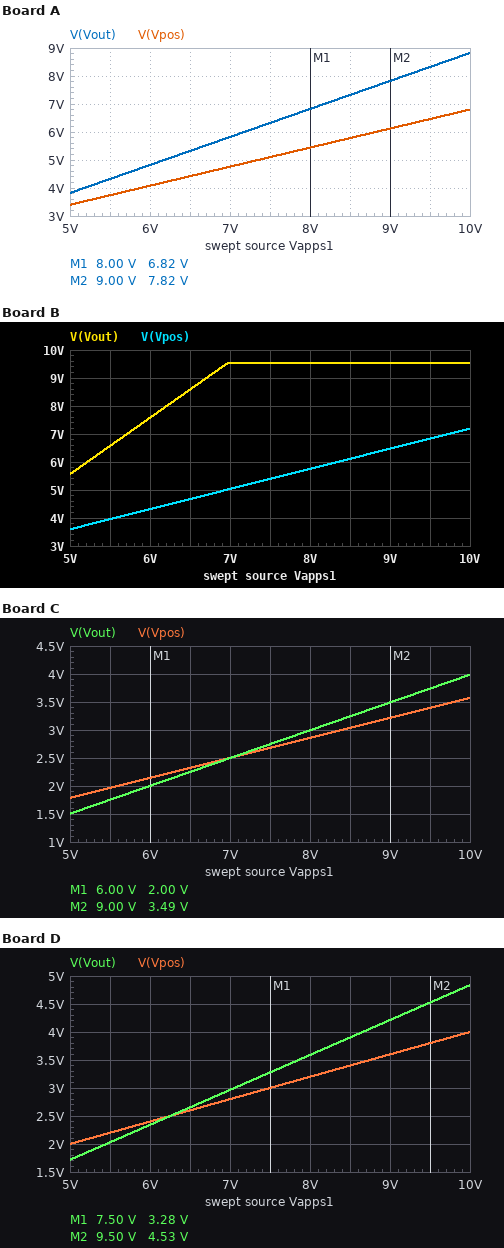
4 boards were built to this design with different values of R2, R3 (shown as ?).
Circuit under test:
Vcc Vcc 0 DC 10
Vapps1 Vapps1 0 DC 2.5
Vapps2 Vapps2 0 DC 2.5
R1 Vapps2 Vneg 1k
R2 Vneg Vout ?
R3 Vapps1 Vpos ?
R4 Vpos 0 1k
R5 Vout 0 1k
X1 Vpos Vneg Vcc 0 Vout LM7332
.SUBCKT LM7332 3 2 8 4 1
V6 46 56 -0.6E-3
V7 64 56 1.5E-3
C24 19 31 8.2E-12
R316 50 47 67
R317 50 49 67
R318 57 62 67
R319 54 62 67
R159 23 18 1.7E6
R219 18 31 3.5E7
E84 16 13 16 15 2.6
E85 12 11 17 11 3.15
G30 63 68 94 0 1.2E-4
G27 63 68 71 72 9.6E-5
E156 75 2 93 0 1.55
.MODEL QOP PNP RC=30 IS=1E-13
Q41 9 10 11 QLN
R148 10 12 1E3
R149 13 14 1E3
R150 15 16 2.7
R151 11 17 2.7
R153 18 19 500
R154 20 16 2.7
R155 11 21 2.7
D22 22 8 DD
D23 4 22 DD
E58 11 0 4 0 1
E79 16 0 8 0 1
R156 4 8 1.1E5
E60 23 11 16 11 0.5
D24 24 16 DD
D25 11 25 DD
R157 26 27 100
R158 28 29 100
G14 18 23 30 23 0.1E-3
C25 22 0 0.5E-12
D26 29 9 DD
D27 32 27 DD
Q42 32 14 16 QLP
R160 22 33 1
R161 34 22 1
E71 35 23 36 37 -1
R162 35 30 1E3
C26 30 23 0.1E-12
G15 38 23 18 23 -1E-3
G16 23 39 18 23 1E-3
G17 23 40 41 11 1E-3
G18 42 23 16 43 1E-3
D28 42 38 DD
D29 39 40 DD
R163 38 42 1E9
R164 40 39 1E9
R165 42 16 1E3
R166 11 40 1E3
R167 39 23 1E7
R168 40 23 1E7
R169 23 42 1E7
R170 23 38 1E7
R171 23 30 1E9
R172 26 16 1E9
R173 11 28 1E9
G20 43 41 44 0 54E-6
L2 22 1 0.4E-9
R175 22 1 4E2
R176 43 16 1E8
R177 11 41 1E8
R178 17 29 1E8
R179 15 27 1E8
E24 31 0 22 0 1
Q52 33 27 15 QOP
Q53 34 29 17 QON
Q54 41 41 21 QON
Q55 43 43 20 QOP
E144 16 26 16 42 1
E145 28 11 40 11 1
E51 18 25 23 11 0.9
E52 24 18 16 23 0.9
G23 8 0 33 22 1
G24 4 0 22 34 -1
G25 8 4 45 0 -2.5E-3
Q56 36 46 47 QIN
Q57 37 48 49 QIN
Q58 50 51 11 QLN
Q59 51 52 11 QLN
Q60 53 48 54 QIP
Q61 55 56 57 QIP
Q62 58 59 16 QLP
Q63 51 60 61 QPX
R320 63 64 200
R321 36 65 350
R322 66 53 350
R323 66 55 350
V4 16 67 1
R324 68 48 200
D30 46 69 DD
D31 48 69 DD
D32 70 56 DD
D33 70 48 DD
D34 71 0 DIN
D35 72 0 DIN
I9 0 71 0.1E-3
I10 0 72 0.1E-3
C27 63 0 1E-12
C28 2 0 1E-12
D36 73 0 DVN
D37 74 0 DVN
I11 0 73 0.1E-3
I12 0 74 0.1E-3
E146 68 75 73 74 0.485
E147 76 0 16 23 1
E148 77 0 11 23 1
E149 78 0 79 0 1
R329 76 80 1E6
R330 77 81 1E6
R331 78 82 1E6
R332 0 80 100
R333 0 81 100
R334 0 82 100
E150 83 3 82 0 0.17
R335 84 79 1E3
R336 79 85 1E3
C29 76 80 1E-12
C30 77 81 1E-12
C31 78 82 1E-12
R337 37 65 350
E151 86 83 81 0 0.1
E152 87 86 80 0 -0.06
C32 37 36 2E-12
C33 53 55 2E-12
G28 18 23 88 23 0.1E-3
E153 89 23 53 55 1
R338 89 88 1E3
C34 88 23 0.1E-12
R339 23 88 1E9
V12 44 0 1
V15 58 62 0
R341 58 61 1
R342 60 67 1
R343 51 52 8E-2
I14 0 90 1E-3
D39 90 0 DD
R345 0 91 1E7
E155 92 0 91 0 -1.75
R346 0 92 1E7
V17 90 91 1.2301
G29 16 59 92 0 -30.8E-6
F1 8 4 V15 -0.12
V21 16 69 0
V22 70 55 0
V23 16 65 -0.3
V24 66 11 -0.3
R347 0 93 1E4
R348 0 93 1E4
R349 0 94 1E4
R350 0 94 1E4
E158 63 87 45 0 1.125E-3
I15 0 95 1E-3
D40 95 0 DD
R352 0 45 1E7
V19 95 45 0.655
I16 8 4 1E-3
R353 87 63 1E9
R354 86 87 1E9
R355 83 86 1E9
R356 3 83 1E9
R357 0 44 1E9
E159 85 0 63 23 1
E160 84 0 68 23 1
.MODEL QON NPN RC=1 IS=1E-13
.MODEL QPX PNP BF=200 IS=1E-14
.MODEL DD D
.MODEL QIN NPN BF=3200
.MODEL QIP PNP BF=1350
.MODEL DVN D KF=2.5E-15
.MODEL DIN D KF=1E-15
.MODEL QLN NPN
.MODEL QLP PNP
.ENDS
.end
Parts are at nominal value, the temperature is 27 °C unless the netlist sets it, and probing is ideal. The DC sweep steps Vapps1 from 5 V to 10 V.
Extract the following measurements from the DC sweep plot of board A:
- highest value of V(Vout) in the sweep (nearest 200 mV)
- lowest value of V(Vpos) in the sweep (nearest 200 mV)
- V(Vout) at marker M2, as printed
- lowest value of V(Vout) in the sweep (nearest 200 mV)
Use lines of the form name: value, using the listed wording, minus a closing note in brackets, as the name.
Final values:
highest value of V(Vout) in the sweep: 8.8 V
lowest value of V(Vpos) in the sweep: 3.4 V
V(Vout) at marker M2, as printed: 7.82 V
lowest value of V(Vout) in the sweep: 3.8 V
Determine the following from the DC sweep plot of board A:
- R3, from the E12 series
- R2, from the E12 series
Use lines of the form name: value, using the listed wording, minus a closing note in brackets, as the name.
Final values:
R3, from the E12 series: 470 Ω
R2, from the E12 series: 470 Ω
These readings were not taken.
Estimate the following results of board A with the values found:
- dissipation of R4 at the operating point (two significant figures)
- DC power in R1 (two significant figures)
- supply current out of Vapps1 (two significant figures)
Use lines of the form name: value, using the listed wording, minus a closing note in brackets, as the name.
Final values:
dissipation of R4 at the operating point: 2.9 mW
DC power in R1: 640 µW
supply current out of Vapps1: 1.7 mA
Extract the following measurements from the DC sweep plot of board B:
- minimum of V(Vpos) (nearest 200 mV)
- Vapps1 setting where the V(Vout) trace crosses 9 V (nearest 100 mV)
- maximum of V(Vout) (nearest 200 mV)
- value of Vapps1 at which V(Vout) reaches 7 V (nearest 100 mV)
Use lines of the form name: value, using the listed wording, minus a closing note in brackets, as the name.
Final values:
minimum of V(Vpos): 3.6 V
Vapps1 setting where the V(Vout) trace crosses 9 V: 6.7 V
maximum of V(Vout): 9.6 V
value of Vapps1 at which V(Vout) reaches 7 V: 5.7 V
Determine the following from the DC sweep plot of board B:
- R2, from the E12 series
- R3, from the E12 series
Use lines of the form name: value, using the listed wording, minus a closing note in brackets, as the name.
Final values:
R2, from the E12 series: 1.8 kΩ
R3, from the E12 series: 390 Ω
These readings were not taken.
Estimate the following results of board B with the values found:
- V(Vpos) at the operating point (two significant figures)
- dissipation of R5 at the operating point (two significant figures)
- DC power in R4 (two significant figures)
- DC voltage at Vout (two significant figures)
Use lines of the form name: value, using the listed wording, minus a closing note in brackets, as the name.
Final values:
V(Vpos) at the operating point: 1.8 V
dissipation of R5 at the operating point: 280 µW
DC power in R4: 3.2 mW
DC voltage at Vout: 530 mV
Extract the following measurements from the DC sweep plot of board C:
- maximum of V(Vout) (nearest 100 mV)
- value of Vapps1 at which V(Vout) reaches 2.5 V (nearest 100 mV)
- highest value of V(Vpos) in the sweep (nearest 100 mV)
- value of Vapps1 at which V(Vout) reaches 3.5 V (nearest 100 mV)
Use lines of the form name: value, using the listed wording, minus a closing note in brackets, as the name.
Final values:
maximum of V(Vout): 4.0 V
value of Vapps1 at which V(Vout) reaches 2.5 V: 7.0 V
highest value of V(Vpos) in the sweep: 3.6 V
value of Vapps1 at which V(Vout) reaches 3.5 V: 9.0 V
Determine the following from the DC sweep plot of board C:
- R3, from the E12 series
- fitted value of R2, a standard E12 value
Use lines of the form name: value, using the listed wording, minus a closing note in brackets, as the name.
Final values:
R3, from the E12 series: 1.8 kΩ
fitted value of R2, a standard E12 value: 390 Ω
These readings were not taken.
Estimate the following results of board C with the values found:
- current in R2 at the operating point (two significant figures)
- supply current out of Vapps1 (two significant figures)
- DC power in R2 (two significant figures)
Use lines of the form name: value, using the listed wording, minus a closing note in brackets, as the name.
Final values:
current in R2 at the operating point: 1.6 mA
supply current out of Vapps1: 890 µA
DC power in R2: 1.0 mW
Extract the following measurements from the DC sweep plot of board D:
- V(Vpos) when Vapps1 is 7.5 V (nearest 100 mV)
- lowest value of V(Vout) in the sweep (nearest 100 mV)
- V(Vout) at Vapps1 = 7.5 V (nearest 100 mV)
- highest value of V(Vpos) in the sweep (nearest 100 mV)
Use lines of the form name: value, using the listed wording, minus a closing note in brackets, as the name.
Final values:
V(Vpos) when Vapps1 is 7.5 V: 3.0 V
lowest value of V(Vout) in the sweep: 1.7 V
V(Vout) at Vapps1 = 7.5 V: 3.3 V
highest value of V(Vpos) in the sweep: 4.0 V
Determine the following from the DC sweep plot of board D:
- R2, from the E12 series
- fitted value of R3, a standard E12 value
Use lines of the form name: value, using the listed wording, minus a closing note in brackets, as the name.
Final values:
R2, from the E12 series: 560 Ω
fitted value of R3, a standard E12 value: 1.5 kΩ
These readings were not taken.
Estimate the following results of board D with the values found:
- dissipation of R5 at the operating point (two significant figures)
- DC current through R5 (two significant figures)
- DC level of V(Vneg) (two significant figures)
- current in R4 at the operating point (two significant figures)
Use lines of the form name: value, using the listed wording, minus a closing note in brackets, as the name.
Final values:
dissipation of R5 at the operating point: 25 µW
DC current through R5: 160 µA
DC level of V(Vneg): 1.0 V
current in R4 at the operating point: 1.0 mA
